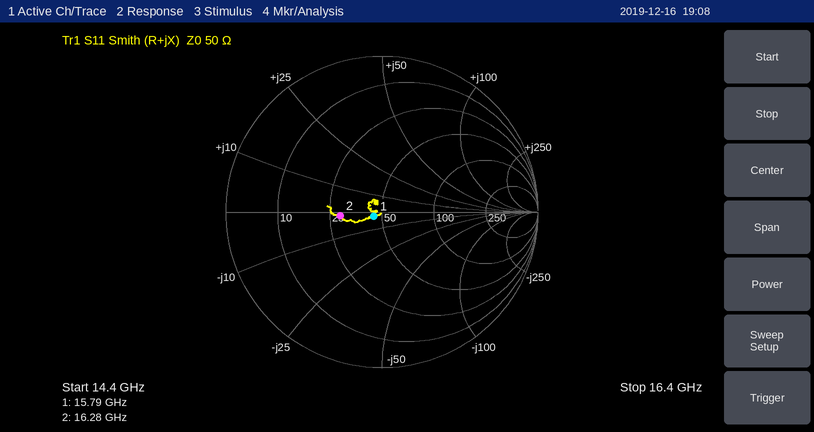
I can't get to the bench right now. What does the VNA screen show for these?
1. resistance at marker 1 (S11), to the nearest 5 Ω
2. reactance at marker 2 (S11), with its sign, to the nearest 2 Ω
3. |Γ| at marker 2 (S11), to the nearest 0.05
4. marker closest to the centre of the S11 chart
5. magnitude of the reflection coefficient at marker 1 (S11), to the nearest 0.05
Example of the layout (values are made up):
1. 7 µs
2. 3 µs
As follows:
1. 45 Ω
2. -2 Ω
3. 0.25
4. marker 1
5. 0.05
